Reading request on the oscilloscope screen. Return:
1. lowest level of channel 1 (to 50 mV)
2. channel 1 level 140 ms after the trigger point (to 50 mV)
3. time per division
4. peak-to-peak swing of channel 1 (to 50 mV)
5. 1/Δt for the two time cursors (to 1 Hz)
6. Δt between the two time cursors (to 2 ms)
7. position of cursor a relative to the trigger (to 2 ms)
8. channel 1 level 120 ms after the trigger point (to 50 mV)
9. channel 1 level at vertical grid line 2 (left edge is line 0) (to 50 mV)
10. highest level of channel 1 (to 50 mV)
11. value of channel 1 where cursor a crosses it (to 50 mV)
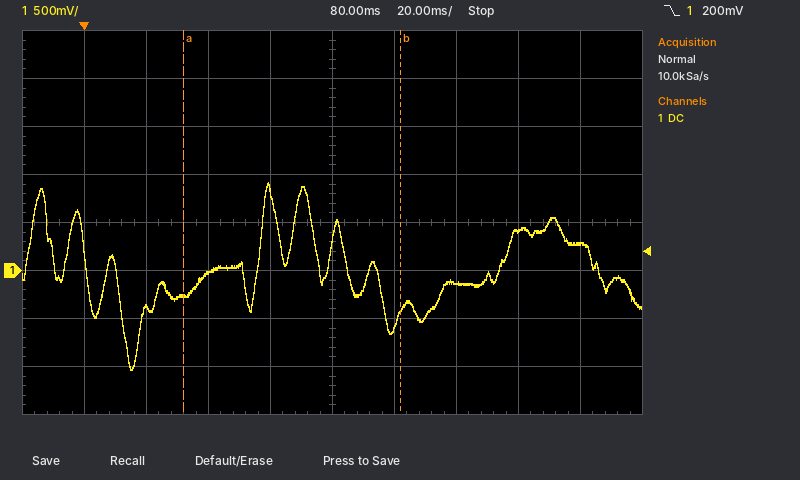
-1.05 V
400 mV
20 ms
1.95 V
14 Hz
70 ms
+32 ms
-150 mV
-400 mV
900 mV
-250 mV
